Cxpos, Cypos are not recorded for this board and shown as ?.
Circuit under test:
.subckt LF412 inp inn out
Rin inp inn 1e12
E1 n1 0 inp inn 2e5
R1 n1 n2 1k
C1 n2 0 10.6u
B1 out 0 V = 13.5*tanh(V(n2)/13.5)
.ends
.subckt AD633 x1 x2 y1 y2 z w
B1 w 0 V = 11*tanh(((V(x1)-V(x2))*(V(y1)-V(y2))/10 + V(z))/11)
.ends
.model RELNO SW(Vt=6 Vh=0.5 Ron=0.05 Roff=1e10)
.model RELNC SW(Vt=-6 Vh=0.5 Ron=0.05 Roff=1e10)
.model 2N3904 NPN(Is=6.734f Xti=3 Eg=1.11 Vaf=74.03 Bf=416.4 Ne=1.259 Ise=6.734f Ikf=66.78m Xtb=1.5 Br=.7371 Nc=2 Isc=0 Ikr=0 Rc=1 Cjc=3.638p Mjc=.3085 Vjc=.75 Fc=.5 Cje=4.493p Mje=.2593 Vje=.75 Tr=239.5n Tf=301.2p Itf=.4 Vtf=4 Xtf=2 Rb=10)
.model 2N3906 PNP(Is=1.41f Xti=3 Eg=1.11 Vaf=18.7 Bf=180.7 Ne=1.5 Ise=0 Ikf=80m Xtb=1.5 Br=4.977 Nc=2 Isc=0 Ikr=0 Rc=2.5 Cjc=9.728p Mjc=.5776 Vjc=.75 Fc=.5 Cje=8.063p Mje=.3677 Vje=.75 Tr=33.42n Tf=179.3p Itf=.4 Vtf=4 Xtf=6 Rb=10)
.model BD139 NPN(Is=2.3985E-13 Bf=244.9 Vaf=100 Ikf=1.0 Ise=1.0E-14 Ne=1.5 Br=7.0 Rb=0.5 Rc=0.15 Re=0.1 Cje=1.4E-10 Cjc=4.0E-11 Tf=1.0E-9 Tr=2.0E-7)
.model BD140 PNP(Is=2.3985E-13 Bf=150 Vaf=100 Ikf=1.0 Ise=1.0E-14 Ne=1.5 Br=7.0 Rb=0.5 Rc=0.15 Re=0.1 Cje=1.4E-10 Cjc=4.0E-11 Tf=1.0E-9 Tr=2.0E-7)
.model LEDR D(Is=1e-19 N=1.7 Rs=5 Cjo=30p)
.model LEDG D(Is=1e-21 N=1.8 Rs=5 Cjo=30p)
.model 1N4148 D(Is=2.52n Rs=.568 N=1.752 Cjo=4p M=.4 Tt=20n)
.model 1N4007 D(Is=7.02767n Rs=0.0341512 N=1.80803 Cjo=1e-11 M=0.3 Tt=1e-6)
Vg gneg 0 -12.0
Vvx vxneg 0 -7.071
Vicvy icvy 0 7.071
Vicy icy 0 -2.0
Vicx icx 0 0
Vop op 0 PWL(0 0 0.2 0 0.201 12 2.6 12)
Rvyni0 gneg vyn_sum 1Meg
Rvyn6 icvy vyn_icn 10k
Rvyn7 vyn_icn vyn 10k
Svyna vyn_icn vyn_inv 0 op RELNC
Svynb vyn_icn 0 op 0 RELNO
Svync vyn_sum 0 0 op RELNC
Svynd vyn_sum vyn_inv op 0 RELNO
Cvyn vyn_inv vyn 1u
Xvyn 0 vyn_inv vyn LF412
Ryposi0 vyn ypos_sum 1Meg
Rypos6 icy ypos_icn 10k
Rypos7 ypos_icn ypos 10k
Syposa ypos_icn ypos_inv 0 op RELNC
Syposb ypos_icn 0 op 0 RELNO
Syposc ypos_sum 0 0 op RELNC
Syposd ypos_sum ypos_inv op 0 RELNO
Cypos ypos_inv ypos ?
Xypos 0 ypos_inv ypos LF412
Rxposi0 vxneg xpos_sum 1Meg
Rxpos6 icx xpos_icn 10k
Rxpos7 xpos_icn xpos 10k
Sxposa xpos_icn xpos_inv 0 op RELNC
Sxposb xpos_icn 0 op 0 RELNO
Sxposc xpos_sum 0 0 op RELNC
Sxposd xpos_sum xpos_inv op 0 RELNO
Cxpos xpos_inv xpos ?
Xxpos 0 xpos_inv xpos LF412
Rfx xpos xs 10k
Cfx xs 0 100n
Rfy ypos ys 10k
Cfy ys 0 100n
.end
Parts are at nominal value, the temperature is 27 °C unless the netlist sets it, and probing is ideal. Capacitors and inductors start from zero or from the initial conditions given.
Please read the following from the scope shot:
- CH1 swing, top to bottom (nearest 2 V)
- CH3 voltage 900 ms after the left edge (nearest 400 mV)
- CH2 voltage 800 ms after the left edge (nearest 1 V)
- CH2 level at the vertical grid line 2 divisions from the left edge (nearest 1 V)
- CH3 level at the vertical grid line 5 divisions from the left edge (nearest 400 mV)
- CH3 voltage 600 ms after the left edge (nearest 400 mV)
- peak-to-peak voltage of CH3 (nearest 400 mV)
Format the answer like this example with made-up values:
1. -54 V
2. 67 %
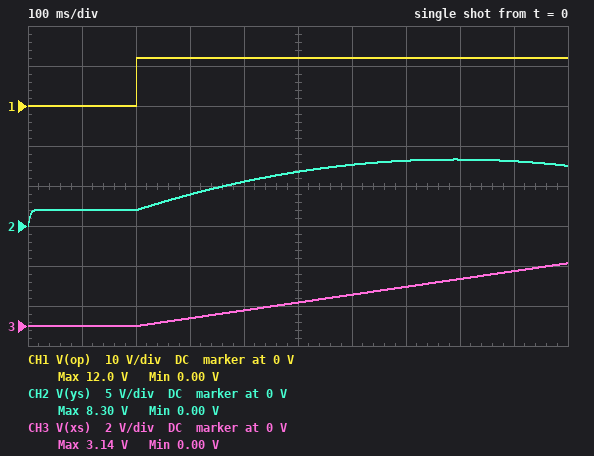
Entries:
1. 12 V
2. 2.8 V
3. 8 V
4. 2 V
5. 1.2 V
6. 1.6 V
7. 3.2 V
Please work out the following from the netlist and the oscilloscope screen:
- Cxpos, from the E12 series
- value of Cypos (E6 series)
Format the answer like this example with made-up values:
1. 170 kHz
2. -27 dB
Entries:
1. 1.8 µF
2. 330 nF
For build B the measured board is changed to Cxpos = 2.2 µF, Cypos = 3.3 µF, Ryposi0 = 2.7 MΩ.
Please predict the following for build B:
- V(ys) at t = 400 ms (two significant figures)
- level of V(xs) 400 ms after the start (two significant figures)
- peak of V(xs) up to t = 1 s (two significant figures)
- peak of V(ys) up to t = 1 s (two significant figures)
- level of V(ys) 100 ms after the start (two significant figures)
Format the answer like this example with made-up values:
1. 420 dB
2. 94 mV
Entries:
1. 2.1 V
2. 640 mV
3. 2.6 V
4. 2.2 V
5. 1.9 V
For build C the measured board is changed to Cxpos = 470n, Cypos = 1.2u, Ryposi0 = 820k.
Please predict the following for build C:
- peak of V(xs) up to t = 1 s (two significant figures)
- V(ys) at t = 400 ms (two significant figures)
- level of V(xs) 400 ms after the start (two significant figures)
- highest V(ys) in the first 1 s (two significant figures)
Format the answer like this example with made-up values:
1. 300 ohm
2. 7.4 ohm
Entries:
1. 12 V
2. 3.2 V
3. 3.0 V
4. 4.1 V
